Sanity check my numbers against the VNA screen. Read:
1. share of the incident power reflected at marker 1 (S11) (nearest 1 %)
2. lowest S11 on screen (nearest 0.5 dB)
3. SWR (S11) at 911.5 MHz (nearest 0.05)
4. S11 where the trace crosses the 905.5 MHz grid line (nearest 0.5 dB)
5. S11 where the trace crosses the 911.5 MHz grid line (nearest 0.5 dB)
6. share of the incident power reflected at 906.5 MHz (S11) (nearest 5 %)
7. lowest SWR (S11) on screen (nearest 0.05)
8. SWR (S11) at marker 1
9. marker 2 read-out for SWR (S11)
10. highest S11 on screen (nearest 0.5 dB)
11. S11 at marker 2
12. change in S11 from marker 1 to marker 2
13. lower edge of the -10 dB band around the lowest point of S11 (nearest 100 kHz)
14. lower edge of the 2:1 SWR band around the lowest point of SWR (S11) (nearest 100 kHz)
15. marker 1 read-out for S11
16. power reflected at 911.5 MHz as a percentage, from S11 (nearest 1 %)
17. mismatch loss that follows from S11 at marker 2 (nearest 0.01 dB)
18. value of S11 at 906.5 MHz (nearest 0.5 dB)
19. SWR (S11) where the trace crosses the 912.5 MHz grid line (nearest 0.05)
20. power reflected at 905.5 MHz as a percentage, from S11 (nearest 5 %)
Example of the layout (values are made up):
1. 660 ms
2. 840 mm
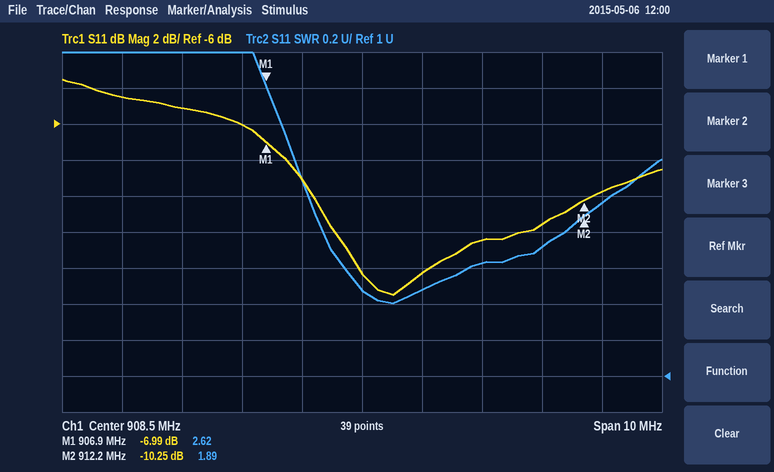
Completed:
1. 20 %
2. -15.5 dB
3. 1.70
4. -5.0 dB
5. -11.5 dB
6. 25 %
7. 1.40
8. 2.62
9. 1.89
10. -3.5 dB
11. -10.25 dB
12. -3.26 dB
13. 907.7 MHz
14. 907.6 MHz
15. -6.99 dB
16. 7 %
17. 0.43 dB
18. -6.0 dB
19. 1.95
20. 30 %
